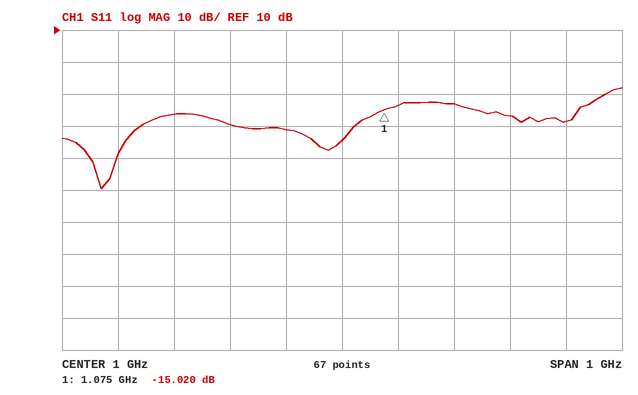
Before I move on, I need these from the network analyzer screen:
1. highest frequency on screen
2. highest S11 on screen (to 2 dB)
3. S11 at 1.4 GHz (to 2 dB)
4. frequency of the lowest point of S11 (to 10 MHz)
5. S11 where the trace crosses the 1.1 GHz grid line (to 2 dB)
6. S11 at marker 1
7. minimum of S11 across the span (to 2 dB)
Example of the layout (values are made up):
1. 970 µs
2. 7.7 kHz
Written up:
1. 1.5 GHz
2. -8 dB
3. -18 dB
4. 570 MHz
5. -14 dB
6. -15.020 dB
7. -40 dB
